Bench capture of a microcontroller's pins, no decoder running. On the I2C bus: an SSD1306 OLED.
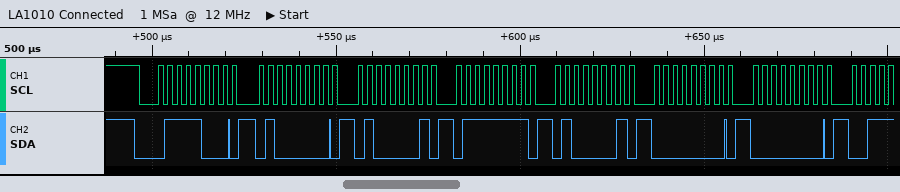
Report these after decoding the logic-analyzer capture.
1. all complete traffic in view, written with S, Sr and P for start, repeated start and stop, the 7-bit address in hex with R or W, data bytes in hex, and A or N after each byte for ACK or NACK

S 3CW A 40 A 41 A 7F A 41 A 00 A 00 A
